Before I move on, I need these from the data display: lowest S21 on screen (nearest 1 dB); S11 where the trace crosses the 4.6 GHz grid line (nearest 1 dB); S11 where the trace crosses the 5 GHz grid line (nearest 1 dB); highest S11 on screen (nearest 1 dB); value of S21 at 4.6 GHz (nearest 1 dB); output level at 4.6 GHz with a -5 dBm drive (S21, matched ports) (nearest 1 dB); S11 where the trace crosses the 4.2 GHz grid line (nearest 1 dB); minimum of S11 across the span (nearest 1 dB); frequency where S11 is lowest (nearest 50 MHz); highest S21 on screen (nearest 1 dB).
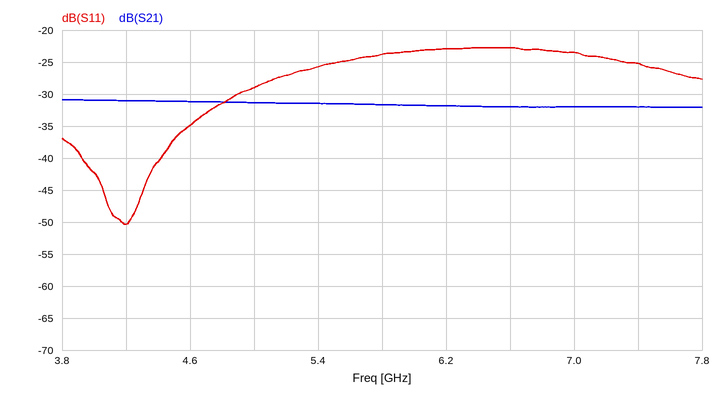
-32 dB
-35 dB
-29 dB
-23 dB
-31 dB
-36 dBm
-50 dB
-50 dB
4.20 GHz
-31 dB
